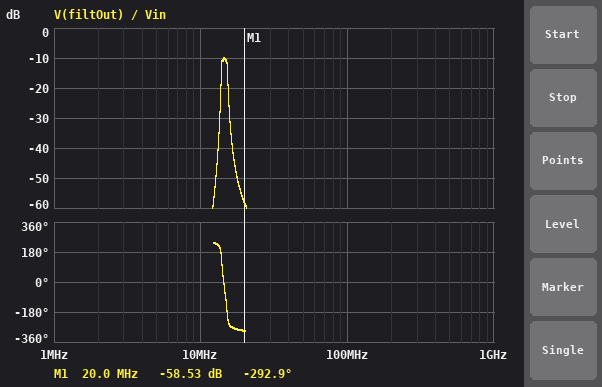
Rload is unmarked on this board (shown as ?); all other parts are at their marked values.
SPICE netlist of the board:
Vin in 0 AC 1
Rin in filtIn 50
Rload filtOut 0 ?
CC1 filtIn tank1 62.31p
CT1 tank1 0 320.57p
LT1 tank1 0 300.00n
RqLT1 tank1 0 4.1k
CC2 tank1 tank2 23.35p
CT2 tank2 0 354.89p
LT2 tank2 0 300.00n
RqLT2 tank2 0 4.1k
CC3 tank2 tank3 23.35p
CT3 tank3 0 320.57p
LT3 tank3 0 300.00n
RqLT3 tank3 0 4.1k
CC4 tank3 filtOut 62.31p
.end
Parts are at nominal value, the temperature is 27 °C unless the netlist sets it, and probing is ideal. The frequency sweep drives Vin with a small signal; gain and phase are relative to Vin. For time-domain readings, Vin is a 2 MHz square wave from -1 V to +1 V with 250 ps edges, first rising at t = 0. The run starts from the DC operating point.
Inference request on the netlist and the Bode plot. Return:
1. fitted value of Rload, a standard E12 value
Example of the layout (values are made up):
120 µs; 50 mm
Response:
33 Ω
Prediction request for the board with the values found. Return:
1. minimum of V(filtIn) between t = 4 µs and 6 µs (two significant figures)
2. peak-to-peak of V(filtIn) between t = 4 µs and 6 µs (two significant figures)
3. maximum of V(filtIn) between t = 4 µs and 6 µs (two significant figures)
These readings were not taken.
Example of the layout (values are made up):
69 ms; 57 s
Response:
-1.1 V; 2.2 V; 1.1 V
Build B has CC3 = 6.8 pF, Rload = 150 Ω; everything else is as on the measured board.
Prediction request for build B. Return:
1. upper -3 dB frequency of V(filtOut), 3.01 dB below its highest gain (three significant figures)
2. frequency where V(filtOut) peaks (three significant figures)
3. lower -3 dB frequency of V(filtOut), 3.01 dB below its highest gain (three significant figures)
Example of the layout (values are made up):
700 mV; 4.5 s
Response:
15.3 MHz; 15.1 MHz; 14.9 MHz
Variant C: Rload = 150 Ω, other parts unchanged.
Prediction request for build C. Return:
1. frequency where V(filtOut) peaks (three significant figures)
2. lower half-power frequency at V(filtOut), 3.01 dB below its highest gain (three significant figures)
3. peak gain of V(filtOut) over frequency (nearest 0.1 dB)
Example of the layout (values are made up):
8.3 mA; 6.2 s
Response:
14.8 MHz; 14.0 MHz; -3.0 dB
